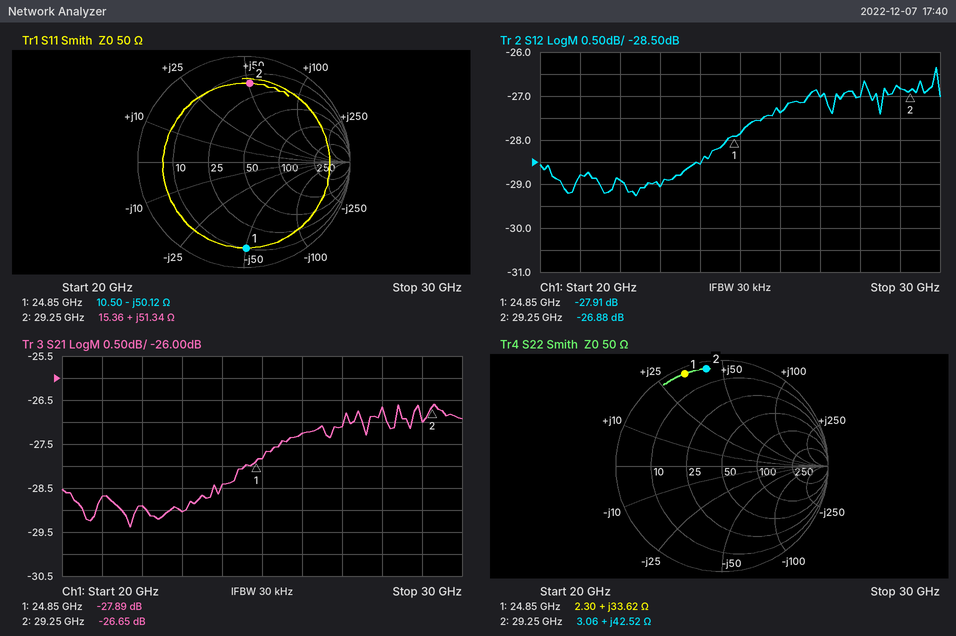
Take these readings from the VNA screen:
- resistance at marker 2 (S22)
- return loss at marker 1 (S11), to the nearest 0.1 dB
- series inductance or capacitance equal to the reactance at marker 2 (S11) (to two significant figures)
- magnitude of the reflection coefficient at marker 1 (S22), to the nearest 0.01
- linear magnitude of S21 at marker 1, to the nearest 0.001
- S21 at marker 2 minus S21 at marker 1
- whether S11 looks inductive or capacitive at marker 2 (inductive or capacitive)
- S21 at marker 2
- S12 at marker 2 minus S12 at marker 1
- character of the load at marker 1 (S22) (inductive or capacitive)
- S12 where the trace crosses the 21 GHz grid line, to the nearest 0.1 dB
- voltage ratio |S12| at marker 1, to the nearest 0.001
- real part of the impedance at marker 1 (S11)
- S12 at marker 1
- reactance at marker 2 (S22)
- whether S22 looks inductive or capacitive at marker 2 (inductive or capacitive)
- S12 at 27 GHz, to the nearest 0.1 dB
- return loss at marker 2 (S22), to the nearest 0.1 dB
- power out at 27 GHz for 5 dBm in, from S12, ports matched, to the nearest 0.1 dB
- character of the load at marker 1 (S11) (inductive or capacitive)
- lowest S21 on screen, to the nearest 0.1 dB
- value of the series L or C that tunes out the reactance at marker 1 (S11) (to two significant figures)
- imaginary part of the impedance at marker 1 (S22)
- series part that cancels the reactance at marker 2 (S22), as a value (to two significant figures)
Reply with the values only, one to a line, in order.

3.06 Ω
1.8 dB
280 pH
0.94
0.040
1.24 dB
inductive
-26.65 dB
1.03 dB
inductive
-28.8 dB
0.040
10.50 Ω
-27.91 dB
+42.52 Ω
inductive
-27.0 dB
0.6 dB
-22.0 dBm
capacitive
-29.4 dB
320 pH
+33.62 Ω
130 fF
